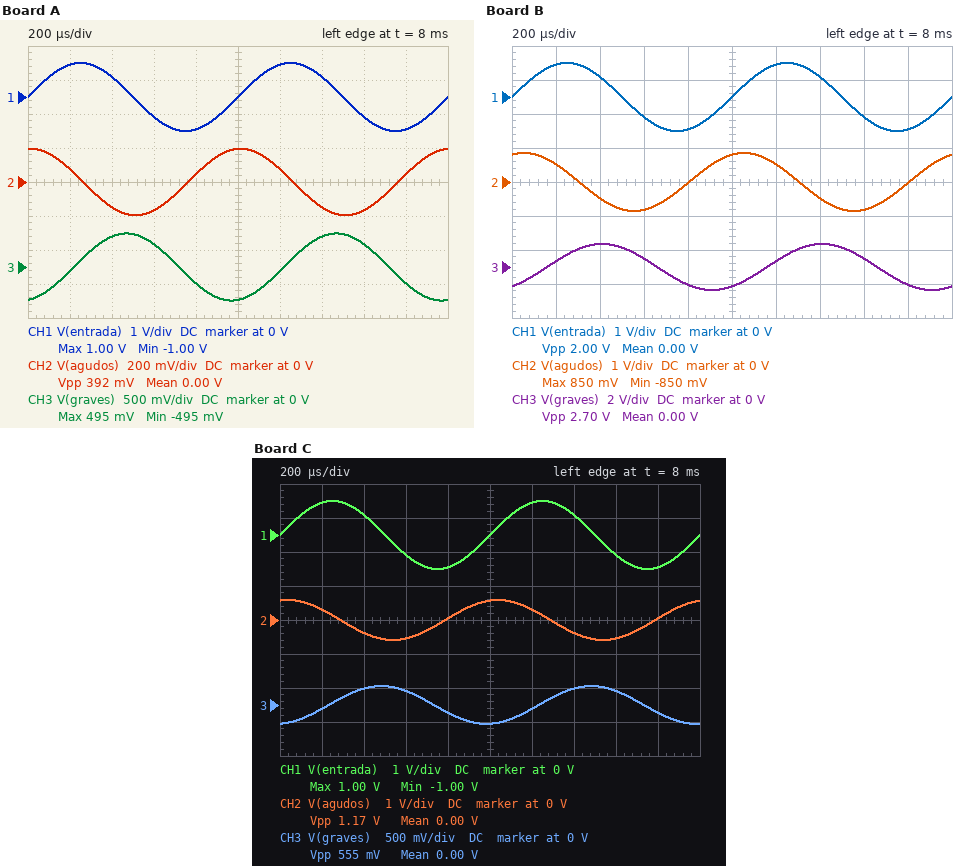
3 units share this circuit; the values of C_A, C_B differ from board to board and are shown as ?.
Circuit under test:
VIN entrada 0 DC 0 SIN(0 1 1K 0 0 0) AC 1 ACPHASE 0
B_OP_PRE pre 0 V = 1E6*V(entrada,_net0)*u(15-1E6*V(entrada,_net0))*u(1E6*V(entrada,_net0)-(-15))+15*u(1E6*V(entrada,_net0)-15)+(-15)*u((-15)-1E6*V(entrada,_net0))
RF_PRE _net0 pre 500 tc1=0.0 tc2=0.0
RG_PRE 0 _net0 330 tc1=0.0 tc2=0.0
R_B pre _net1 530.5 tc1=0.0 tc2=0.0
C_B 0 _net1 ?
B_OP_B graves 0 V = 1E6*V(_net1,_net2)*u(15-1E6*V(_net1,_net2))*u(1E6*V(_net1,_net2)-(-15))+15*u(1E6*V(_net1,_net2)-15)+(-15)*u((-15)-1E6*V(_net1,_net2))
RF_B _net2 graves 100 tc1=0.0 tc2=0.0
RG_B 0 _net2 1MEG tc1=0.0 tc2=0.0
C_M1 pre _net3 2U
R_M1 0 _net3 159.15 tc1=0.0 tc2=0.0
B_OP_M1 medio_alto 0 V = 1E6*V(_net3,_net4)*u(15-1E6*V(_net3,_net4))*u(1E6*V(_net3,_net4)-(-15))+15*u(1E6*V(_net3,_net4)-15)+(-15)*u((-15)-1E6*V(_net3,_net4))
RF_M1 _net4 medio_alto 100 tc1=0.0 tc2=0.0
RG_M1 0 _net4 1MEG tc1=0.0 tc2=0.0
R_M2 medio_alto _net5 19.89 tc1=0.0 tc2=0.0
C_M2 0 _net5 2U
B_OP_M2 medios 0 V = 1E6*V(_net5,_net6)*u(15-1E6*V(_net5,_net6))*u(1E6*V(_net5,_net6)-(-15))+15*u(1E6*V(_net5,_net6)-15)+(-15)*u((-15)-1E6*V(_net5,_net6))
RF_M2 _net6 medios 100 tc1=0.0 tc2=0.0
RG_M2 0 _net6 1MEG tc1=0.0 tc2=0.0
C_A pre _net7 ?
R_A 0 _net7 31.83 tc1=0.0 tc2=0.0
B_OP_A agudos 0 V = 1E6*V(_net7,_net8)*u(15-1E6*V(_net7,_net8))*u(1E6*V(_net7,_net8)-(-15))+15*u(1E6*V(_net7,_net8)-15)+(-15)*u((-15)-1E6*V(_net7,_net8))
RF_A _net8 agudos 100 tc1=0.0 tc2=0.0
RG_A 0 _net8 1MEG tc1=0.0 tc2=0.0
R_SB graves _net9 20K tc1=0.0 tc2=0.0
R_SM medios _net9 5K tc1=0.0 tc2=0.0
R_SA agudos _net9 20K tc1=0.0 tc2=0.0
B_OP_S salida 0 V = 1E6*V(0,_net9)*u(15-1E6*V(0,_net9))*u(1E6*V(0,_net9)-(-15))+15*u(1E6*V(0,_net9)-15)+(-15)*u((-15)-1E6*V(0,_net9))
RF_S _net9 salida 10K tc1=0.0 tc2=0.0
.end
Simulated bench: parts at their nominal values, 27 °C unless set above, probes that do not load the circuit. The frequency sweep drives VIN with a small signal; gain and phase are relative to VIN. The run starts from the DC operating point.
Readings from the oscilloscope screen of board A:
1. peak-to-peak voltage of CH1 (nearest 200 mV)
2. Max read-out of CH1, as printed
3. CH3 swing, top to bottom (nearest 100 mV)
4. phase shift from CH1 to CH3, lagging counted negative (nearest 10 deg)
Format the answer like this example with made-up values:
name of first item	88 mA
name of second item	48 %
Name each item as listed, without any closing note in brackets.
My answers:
peak-to-peak voltage of CH1	2.0 V
Max read-out of CH1, as printed	1.00 V
CH3 swing, top to bottom	1.0 V
phase shift from CH1 to CH3, lagging counted negative	-80 deg
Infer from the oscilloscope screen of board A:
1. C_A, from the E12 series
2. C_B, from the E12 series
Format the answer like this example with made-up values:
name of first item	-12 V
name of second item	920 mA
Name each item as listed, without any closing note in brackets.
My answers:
C_A, from the E12 series	390 nF
C_B, from the E12 series	1.5 µF
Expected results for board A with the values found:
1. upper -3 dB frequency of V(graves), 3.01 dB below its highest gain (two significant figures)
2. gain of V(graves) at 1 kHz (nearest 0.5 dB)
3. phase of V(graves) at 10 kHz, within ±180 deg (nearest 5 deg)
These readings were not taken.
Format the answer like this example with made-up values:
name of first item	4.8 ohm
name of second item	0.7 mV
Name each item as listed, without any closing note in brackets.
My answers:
upper -3 dB frequency of V(graves), 3.01 dB below its highest gain	200 Hz
gain of V(graves) at 1 kHz	-6.0 dB
phase of V(graves) at 10 kHz, within ±180 deg	-90 deg
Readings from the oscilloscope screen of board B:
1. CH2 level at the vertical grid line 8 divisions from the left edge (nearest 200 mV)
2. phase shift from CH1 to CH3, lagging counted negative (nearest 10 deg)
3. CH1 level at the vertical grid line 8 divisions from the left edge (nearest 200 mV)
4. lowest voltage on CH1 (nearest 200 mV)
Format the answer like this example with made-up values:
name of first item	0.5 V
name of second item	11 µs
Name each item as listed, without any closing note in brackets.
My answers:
CH2 level at the vertical grid line 8 divisions from the left edge	-800 mV
phase shift from CH1 to CH3, lagging counted negative	-60 deg
CH1 level at the vertical grid line 8 divisions from the left edge	-600 mV
lowest voltage on CH1	-1.0 V
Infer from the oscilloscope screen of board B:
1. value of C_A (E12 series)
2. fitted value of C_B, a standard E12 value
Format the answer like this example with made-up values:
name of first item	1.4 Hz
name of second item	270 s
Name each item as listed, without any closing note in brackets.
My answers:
value of C_A	1.8 µF
fitted value of C_B, a standard E12 value	470 nF
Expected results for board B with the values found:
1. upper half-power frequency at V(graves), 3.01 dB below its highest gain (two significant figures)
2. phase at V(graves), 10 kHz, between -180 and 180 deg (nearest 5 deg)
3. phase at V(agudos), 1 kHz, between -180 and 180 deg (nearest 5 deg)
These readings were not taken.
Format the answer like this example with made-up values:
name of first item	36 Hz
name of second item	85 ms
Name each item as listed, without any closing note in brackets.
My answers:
upper half-power frequency at V(graves), 3.01 dB below its highest gain	640 Hz
phase at V(graves), 10 kHz, between -180 and 180 deg	-85 deg
phase at V(agudos), 1 kHz, between -180 and 180 deg	70 deg
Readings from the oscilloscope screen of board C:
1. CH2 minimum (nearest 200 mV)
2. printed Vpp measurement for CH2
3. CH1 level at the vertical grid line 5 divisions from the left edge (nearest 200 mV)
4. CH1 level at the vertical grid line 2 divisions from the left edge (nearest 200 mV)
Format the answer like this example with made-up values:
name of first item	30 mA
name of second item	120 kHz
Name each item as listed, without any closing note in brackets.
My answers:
CH2 minimum	-600 mV
printed Vpp measurement for CH2	1.17 V
CH1 level at the vertical grid line 5 divisions from the left edge	0 V
CH1 level at the vertical grid line 2 divisions from the left edge	600 mV
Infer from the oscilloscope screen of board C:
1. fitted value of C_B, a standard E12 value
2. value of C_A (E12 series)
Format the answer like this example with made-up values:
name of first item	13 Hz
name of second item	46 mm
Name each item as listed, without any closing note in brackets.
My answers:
fitted value of C_B, a standard E12 value	2.7 µF
value of C_A	1.2 µF
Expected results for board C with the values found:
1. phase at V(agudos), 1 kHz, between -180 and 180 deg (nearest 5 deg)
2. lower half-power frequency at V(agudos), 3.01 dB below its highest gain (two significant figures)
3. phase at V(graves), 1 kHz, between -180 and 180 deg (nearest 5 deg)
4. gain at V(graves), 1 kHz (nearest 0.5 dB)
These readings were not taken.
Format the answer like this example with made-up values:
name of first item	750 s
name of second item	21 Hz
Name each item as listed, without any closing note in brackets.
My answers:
phase at V(agudos), 1 kHz, between -180 and 180 deg	75 deg
lower half-power frequency at V(agudos), 3.01 dB below its highest gain	4.2 kHz
phase at V(graves), 1 kHz, between -180 and 180 deg	-85 deg
gain at V(graves), 1 kHz	-11.0 dB
